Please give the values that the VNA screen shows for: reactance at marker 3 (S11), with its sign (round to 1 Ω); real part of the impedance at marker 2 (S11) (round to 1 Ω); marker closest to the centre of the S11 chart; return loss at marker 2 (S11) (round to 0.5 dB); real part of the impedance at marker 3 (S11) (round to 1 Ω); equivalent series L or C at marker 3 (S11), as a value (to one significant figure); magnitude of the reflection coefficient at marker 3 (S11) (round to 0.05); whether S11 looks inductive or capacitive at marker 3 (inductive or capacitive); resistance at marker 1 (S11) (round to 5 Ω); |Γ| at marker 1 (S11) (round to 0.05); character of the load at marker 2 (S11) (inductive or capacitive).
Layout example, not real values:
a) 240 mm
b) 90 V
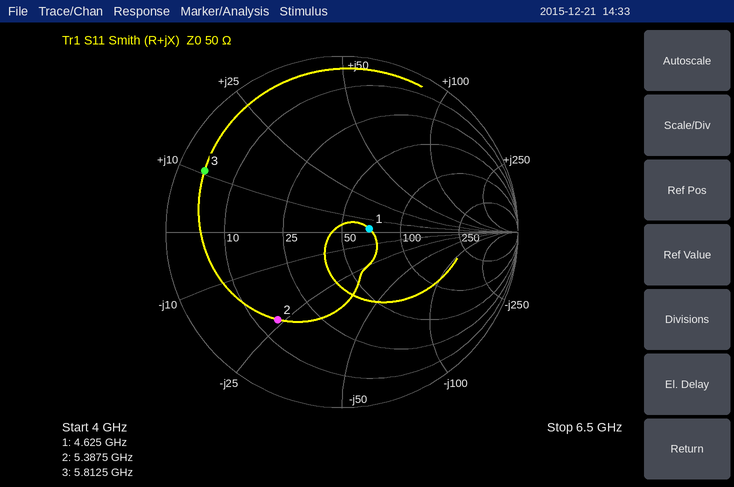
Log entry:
a) +11 Ω
b) 15 Ω
c) marker 1
d) 4.0 dB
e) 4 Ω
f) 300 pH
g) 0.85
h) inductive
i) 70 Ω
j) 0.15
k) capacitive
